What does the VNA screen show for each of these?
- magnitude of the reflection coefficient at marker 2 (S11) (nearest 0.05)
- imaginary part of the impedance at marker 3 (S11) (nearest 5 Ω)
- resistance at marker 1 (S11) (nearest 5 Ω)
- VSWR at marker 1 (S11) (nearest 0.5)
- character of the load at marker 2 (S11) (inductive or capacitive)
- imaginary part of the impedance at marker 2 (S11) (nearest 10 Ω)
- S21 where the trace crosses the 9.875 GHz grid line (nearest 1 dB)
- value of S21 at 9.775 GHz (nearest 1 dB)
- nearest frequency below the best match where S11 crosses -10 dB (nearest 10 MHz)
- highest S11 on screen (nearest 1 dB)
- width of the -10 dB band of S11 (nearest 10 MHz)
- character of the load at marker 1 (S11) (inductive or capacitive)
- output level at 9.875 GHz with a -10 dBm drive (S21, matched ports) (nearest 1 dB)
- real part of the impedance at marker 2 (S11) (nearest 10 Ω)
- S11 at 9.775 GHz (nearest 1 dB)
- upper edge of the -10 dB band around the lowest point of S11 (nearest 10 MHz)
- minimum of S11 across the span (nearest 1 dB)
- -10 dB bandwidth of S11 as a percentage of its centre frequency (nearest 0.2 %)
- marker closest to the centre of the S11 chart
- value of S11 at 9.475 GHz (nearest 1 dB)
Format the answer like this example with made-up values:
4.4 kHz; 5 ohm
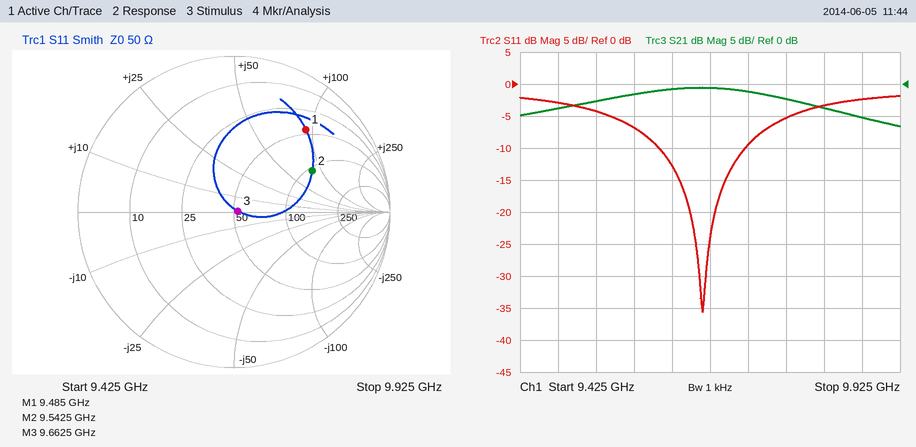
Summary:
0.55; 0 Ω; 45 Ω; 5.5; inductive; +80 Ω; -5 dB; -2 dB; 9.61 GHz; -2 dB; 110 MHz; inductive; -15 dBm; 110 Ω; -5 dB; 9.72 GHz; -36 dB; 1.2 %; marker 3; -3 dB
